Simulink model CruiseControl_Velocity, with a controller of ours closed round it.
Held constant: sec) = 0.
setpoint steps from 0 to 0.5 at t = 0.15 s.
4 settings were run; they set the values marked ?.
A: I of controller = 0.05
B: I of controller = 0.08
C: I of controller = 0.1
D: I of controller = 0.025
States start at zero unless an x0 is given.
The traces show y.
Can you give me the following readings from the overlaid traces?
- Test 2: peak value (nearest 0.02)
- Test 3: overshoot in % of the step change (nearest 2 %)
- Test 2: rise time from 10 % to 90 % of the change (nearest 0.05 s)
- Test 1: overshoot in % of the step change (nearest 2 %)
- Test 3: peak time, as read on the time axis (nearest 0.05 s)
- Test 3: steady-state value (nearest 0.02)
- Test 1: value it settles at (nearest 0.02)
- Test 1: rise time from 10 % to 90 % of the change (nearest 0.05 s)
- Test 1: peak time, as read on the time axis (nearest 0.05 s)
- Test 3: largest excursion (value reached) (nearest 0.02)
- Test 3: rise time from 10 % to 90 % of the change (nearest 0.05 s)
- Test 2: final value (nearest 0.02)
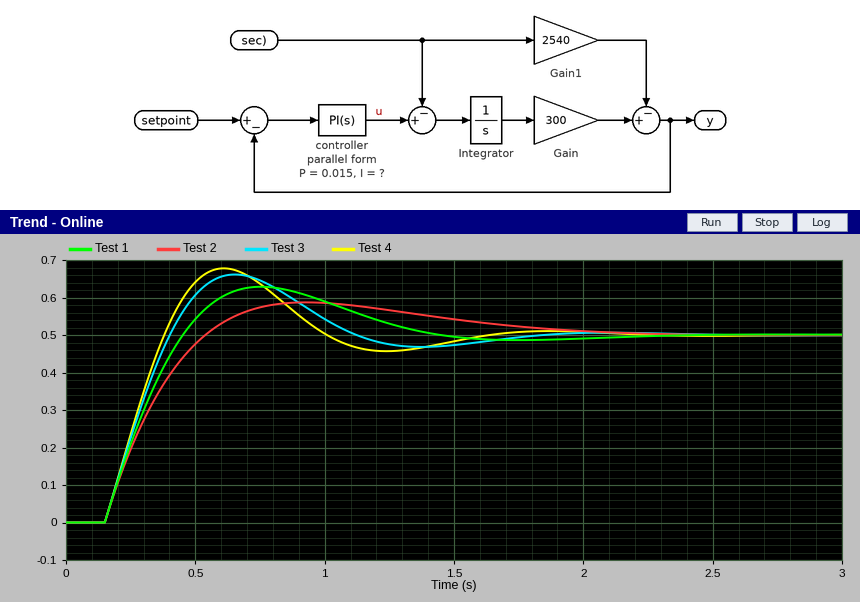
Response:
0.58
32 %
0.30 s
26 %
0.65 s
0.50
0.50
0.25 s
0.75 s
0.66
0.20 s
0.50
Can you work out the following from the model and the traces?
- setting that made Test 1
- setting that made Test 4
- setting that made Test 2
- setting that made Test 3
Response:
A
C
D
B
